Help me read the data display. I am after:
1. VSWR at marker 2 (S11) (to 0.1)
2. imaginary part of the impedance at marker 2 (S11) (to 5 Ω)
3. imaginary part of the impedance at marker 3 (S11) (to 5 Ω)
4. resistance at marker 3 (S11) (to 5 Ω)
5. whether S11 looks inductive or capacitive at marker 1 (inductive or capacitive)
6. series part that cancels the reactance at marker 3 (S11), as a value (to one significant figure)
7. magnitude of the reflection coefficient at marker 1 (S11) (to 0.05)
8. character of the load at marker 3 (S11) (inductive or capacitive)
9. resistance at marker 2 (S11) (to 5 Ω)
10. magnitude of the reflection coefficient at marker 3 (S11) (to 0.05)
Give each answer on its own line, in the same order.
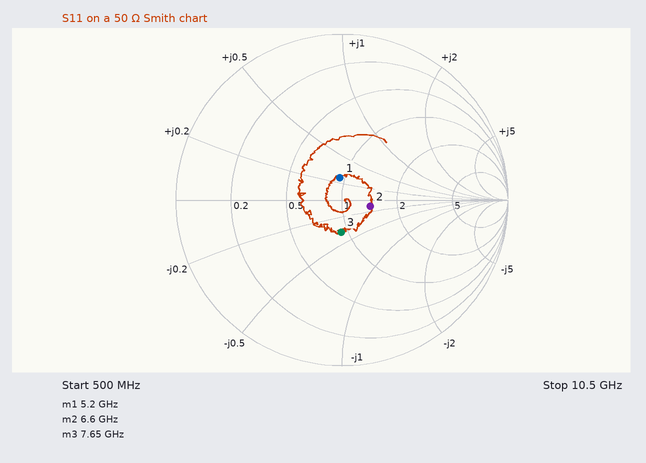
1.4
-5 Ω
-20 Ω
45 Ω
inductive
400 pH
0.15
capacitive
70 Ω
0.20
